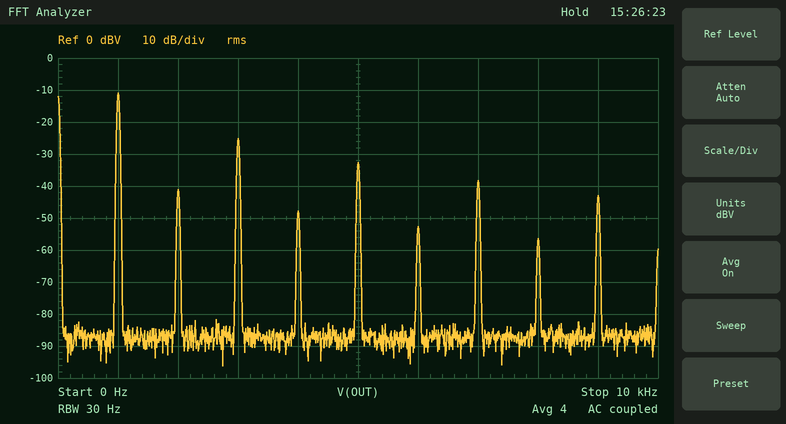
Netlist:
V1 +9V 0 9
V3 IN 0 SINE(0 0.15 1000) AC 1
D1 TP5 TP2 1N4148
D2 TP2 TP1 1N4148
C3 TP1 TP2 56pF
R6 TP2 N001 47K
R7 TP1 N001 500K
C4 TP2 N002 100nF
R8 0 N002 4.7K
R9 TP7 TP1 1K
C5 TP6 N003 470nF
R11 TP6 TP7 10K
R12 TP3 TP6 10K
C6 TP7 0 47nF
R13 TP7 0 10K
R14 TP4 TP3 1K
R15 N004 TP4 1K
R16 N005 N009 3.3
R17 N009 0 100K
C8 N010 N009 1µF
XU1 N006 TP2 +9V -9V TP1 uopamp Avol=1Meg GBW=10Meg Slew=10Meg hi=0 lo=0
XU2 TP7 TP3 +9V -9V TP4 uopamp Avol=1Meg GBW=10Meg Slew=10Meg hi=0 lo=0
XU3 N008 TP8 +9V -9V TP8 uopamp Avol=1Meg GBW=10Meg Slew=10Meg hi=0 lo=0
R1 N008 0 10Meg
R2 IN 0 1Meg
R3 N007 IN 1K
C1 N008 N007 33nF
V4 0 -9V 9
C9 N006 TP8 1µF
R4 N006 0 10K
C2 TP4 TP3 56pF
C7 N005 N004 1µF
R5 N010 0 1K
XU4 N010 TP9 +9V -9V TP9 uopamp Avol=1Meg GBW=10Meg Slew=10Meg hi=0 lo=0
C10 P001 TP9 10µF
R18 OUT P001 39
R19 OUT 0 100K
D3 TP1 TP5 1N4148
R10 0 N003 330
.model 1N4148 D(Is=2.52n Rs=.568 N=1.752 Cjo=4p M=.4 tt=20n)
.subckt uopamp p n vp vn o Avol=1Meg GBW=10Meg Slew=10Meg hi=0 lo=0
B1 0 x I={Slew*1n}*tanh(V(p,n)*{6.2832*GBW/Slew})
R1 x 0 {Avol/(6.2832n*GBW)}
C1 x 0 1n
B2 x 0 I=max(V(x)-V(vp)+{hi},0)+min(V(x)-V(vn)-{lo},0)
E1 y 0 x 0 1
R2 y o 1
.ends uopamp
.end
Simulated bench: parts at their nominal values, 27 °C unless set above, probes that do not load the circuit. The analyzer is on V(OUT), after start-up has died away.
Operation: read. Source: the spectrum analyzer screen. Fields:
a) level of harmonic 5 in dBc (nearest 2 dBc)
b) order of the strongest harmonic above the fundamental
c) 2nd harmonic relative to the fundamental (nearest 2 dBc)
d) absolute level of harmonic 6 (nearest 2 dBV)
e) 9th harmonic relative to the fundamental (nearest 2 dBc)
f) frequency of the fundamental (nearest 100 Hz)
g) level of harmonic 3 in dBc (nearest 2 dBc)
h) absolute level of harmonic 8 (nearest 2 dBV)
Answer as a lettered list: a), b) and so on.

a) -22 dBc
b) 3
c) -30 dBc
d) -52 dBV
e) -32 dBc
f) 1.0 kHz
g) -14 dBc
h) -56 dBV
